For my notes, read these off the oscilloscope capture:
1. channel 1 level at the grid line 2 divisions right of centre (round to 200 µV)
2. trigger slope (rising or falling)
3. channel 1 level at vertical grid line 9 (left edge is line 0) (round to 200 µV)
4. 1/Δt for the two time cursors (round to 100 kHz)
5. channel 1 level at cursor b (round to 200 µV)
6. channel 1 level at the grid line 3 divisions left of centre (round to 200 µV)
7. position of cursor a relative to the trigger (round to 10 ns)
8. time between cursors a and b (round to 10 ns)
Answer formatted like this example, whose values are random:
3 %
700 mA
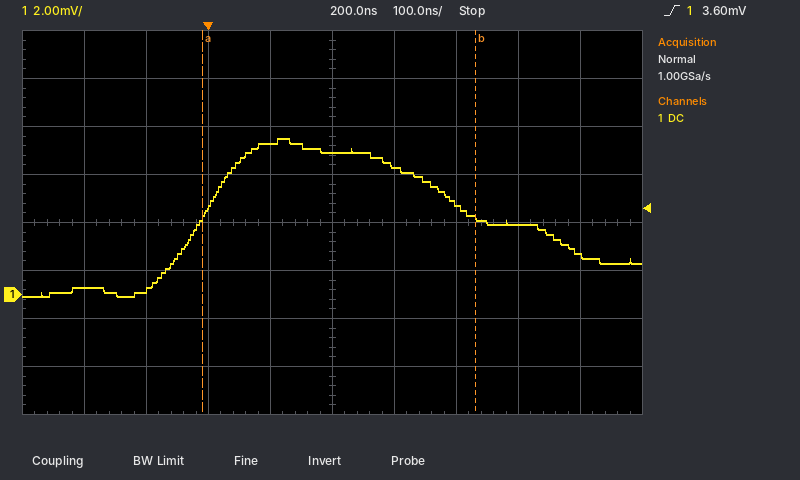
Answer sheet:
3.8 mV
rising
1.6 mV
2.3 MHz
3.2 mV
200 µV
-10 ns
440 ns
